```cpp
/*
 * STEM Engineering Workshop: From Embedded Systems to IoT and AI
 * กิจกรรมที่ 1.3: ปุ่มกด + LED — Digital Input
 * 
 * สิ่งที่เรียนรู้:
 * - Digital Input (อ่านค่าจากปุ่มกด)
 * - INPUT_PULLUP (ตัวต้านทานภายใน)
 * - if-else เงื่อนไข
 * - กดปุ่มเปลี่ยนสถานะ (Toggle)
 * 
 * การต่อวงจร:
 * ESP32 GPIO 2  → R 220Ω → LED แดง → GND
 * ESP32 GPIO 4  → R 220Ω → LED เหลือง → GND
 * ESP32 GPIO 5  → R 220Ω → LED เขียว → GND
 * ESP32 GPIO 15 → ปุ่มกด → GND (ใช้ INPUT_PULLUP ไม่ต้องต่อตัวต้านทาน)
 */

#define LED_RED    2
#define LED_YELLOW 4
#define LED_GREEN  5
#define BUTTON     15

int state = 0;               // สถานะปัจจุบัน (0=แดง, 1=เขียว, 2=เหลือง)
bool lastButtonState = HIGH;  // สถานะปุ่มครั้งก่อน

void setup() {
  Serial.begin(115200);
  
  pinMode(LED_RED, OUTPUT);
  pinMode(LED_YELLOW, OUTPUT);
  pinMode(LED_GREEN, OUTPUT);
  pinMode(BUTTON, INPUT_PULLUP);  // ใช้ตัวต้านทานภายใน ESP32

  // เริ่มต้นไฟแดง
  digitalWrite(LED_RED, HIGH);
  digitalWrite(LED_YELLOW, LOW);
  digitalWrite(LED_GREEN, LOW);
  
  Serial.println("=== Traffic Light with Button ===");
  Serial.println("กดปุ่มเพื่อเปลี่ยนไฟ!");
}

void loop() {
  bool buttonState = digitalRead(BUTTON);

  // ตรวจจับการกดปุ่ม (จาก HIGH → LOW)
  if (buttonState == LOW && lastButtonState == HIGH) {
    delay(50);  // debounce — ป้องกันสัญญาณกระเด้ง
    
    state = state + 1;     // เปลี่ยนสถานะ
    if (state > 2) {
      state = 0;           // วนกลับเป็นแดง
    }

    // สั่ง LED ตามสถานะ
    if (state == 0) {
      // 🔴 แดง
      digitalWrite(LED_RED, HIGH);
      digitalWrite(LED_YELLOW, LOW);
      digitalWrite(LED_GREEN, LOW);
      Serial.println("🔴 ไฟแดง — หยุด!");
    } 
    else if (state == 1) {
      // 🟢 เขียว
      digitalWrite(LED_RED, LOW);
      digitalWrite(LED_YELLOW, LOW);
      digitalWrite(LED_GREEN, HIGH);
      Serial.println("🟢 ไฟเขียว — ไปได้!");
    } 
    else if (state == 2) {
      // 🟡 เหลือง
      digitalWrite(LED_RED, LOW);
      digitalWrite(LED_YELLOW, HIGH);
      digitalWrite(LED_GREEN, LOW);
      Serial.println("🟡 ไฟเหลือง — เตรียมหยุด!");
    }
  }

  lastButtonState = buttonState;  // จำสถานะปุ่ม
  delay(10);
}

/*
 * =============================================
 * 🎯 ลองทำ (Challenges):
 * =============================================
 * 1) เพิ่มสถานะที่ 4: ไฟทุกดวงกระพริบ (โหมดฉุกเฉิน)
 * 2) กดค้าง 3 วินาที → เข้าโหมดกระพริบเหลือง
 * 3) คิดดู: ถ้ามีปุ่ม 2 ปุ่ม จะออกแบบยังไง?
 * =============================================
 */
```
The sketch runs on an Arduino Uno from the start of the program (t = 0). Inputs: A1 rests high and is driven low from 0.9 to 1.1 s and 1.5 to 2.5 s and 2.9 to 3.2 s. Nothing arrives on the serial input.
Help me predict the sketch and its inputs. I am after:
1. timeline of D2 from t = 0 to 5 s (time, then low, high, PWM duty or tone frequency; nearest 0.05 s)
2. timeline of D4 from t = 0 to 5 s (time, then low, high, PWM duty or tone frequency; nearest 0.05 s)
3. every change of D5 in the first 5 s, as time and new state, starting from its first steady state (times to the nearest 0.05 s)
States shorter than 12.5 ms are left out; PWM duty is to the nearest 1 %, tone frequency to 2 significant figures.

0 s high; 0.95 s low; 2.95 s high
0 s low; 1.55 s high; 2.95 s low
0 s low; 0.95 s high; 1.55 s low
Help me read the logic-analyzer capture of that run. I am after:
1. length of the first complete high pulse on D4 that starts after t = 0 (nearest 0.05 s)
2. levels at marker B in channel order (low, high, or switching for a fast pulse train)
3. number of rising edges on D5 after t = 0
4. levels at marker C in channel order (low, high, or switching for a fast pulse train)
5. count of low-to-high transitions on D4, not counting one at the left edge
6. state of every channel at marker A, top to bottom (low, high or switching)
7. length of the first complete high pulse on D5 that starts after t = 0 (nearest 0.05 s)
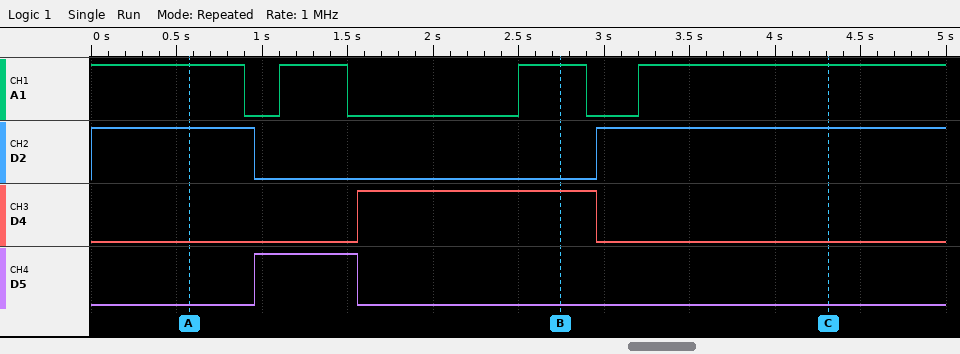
1.40 s
A1 high, D2 low, D4 high, D5 low
1
A1 high, D2 high, D4 low, D5 low
1
A1 high, D2 high, D4 low, D5 low
0.60 s
